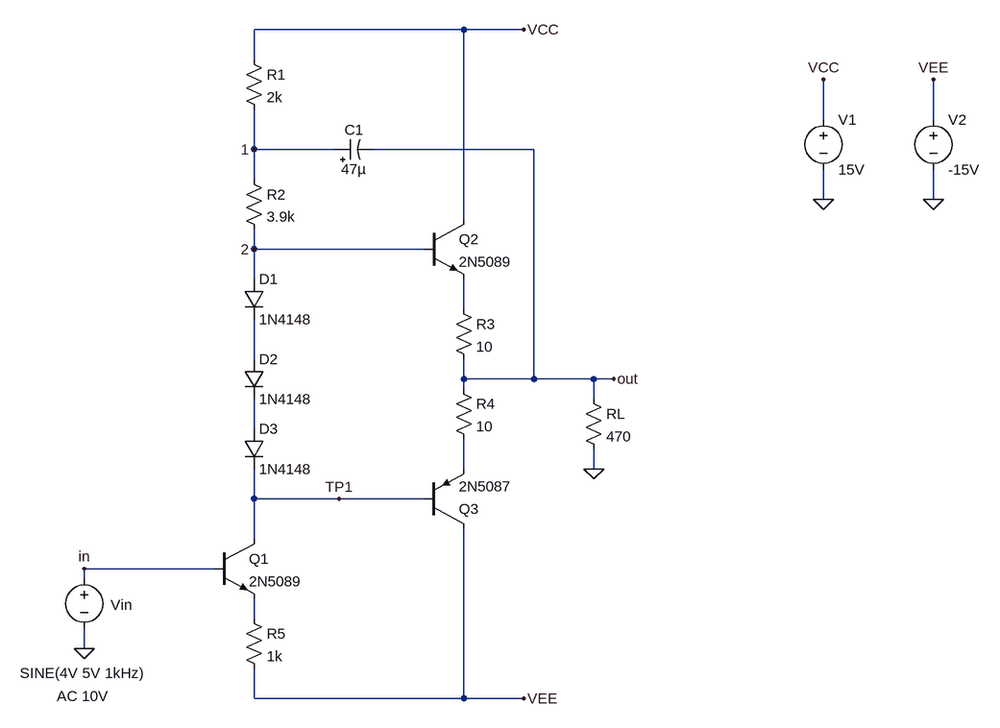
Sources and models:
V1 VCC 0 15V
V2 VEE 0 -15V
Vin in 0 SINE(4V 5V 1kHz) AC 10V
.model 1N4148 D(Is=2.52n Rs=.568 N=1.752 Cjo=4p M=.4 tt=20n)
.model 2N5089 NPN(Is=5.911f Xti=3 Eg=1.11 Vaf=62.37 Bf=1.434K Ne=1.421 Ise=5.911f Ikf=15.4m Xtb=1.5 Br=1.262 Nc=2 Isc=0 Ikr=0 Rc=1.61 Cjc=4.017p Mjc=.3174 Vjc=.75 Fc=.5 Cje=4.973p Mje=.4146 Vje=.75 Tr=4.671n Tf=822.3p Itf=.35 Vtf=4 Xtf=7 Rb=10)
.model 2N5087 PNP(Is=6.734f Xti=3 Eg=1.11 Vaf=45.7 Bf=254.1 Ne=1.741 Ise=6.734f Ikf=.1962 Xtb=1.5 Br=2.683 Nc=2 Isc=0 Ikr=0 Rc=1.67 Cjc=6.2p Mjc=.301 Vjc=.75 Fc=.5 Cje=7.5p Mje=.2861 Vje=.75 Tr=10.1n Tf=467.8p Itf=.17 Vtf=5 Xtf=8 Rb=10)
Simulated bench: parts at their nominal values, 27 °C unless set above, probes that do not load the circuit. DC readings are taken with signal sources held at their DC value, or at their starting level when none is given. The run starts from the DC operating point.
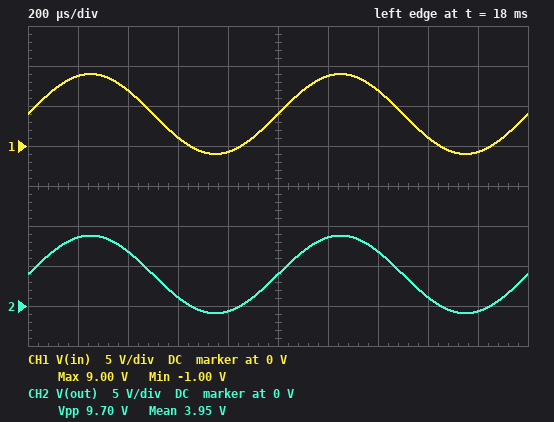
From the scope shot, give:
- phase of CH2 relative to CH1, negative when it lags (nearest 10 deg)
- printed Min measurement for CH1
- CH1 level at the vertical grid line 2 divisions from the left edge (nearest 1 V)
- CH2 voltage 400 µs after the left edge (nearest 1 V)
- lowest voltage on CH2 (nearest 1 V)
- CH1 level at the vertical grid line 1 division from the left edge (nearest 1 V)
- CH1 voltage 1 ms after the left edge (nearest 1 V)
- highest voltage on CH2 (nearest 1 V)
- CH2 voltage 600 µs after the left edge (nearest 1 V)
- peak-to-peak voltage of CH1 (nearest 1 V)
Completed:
0 deg
-1.00 V
7 V
7 V
-1 V
9 V
4 V
9 V
1 V
10 V
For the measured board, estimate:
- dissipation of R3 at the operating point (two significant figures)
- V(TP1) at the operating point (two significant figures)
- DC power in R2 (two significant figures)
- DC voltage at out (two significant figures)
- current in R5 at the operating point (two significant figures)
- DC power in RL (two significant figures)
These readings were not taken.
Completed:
4.4 mW
3.1 V
11 mW
3.9 V
18 mA
33 mW
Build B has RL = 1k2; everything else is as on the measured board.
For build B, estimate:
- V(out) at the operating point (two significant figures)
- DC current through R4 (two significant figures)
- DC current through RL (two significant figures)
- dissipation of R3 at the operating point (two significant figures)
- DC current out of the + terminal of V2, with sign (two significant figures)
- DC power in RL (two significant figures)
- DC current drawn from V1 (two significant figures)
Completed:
4.0 V
15 mA
3.3 mA
3.4 mW
-33 mA
13 mW
20 mA
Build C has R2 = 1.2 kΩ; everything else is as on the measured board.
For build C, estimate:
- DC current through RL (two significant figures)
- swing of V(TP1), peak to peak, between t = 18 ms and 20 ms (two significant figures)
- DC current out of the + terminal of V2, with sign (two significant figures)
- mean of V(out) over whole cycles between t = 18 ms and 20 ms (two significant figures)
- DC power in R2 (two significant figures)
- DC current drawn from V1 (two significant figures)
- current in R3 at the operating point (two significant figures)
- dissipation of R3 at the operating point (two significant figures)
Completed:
8.5 mA
9.9 V
-34 mA
4.0 V
12 mW
28 mA
25 mA
6.1 mW
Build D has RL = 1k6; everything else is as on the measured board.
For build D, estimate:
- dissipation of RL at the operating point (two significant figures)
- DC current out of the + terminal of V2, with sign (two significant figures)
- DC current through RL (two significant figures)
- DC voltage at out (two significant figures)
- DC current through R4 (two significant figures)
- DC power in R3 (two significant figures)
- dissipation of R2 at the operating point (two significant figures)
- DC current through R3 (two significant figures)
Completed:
9.9 mW
-34 mA
2.5 mA
4.0 V
16 mA
3.3 mW
11 mW
18 mA
